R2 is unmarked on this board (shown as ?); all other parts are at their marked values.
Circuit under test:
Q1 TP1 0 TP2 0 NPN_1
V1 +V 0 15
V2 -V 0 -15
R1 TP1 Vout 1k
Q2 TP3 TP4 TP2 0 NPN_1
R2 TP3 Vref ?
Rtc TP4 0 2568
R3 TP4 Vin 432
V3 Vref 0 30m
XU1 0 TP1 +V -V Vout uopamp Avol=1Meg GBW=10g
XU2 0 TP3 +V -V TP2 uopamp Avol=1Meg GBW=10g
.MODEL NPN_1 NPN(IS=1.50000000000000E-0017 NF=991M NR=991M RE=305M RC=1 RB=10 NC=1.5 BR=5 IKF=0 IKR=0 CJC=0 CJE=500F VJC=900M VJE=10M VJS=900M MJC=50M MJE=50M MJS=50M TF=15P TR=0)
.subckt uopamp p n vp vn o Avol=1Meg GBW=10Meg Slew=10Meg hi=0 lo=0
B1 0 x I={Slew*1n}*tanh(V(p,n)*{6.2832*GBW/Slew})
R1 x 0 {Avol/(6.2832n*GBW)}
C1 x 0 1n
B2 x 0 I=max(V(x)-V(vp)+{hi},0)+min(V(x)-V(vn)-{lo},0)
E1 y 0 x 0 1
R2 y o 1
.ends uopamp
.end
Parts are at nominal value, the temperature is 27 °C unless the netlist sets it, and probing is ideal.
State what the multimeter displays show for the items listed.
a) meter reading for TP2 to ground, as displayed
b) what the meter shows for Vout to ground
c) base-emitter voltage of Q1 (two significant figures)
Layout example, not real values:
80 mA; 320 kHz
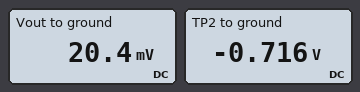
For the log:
-0.716 V; 20.4 mV; 720 mV
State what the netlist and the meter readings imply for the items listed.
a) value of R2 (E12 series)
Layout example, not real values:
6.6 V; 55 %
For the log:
1.5 kΩ
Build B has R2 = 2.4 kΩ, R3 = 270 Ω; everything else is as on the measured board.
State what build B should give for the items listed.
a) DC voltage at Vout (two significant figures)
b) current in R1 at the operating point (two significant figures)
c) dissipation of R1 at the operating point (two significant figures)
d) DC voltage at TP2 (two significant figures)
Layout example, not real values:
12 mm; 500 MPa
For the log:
13 mV; 13 µA; 160 nW; -700 mV
